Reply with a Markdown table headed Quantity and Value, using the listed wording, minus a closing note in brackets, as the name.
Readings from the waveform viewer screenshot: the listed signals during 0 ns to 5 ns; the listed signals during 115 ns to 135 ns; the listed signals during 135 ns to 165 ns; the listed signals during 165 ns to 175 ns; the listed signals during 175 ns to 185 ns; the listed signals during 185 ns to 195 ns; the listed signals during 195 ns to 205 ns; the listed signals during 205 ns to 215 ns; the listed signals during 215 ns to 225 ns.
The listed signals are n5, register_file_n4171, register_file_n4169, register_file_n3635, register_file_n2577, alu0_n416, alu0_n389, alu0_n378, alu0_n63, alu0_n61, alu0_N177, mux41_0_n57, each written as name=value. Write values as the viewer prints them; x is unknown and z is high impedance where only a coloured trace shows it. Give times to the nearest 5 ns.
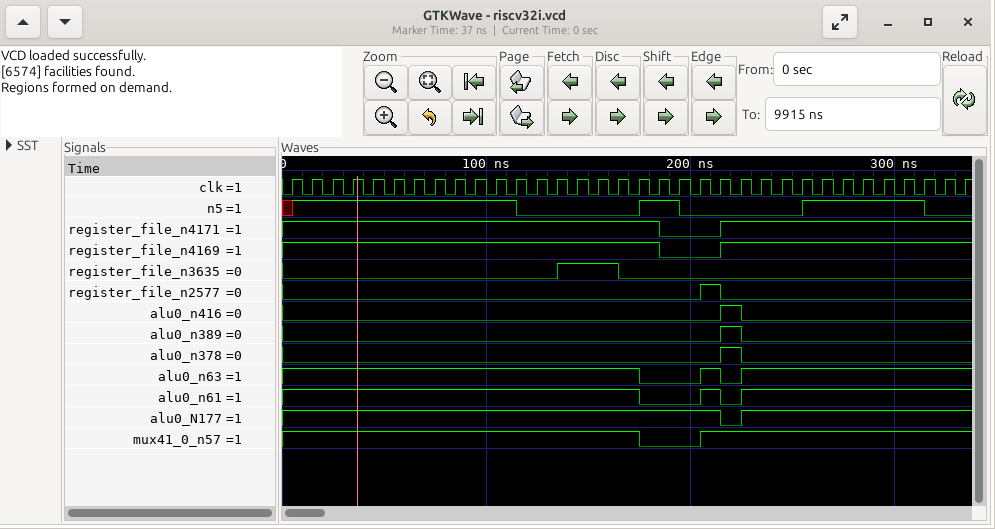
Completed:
| Quantity | Value |
|---|---|
| the listed signals during 0 ns to 5 ns | n5=x, register_file_n4171=1, register_file_n4169=1, register_file_n3635=0, register_file_n2577=0, alu0_n416=0, alu0_n389=0, alu0_n378=0, alu0_n63=1, alu0_n61=1, alu0_N177=1, mux41_0_n57=1 |
| the listed signals during 115 ns to 135 ns | n5=0, register_file_n4171=1, register_file_n4169=1, register_file_n3635=0, register_file_n2577=0, alu0_n416=0, alu0_n389=0, alu0_n378=0, alu0_n63=1, alu0_n61=1, alu0_N177=1, mux41_0_n57=1 |
| the listed signals during 135 ns to 165 ns | n5=0, register_file_n4171=1, register_file_n4169=1, register_file_n3635=1, register_file_n2577=0, alu0_n416=0, alu0_n389=0, alu0_n378=0, alu0_n63=1, alu0_n61=1, alu0_N177=1, mux41_0_n57=1 |
| the listed signals during 165 ns to 175 ns | n5=0, register_file_n4171=1, register_file_n4169=1, register_file_n3635=0, register_file_n2577=0, alu0_n416=0, alu0_n389=0, alu0_n378=0, alu0_n63=1, alu0_n61=1, alu0_N177=1, mux41_0_n57=1 |
| the listed signals during 175 ns to 185 ns | n5=1, register_file_n4171=1, register_file_n4169=1, register_file_n3635=0, register_file_n2577=0, alu0_n416=0, alu0_n389=0, alu0_n378=0, alu0_n63=0, alu0_n61=0, alu0_N177=1, mux41_0_n57=0 |
| the listed signals during 185 ns to 195 ns | n5=1, register_file_n4171=0, register_file_n4169=0, register_file_n3635=0, register_file_n2577=0, alu0_n416=0, alu0_n389=0, alu0_n378=0, alu0_n63=0, alu0_n61=0, alu0_N177=1, mux41_0_n57=0 |
| the listed signals during 195 ns to 205 ns | n5=0, register_file_n4171=0, register_file_n4169=0, register_file_n3635=0, register_file_n2577=0, alu0_n416=0, alu0_n389=0, alu0_n378=0, alu0_n63=0, alu0_n61=0, alu0_N177=1, mux41_0_n57=0 |
| the listed signals during 205 ns to 215 ns | n5=0, register_file_n4171=0, register_file_n4169=0, register_file_n3635=0, register_file_n2577=1, alu0_n416=0, alu0_n389=0, alu0_n378=0, alu0_n63=1, alu0_n61=1, alu0_N177=1, mux41_0_n57=1 |
| the listed signals during 215 ns to 225 ns | n5=0, register_file_n4171=1, register_file_n4169=1, register_file_n3635=0, register_file_n2577=0, alu0_n416=1, alu0_n389=1, alu0_n378=1, alu0_n63=0, alu0_n61=0, alu0_N177=0, mux41_0_n57=1 |
